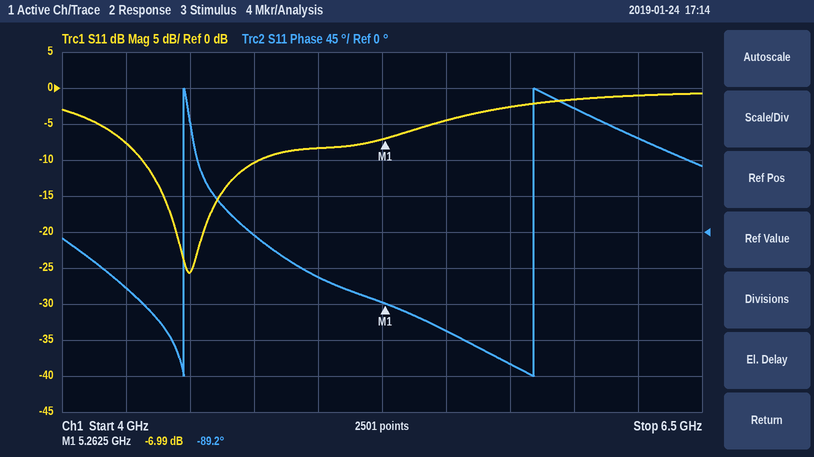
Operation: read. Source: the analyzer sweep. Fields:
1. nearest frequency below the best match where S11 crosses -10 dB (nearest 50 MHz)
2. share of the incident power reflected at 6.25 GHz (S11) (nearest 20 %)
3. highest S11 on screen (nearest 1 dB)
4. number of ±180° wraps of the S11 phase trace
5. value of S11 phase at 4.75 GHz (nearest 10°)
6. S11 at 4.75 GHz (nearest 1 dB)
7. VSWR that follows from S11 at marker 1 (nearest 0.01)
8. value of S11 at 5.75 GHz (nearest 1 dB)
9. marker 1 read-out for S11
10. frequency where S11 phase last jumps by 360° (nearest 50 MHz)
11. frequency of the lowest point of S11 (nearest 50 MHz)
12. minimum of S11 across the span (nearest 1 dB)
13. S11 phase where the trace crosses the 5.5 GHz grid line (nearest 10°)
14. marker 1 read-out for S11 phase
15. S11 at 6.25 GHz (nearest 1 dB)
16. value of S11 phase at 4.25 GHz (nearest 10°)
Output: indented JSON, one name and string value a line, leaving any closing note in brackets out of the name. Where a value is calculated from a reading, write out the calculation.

{
  "nearest frequency below the best match where S11 crosses -10 dB": "4.30 GHz",
  "share of the incident power reflected at 6.25 GHz (S11)": "10^(-1/10) ≈ 79.4 %, so 80 % to the nearest 20 %",
  "highest S11 on screen": "-1 dB",
  "number of ±180° wraps of the S11 phase trace": "2",
  "value of S11 phase at 4.75 GHz": "0°",
  "S11 at 4.75 GHz": "-10 dB",
  "VSWR that follows from S11 at marker 1": "(1 + 0.4472)/(1 − 0.4472) ≈ 2.62",
  "value of S11 at 5.75 GHz": "-3 dB",
  "marker 1 read-out for S11": "-6.99 dB",
  "frequency where S11 phase last jumps by 360°": "5.85 GHz",
  "frequency of the lowest point of S11": "4.50 GHz",
  "minimum of S11 across the span": "-26 dB",
  "S11 phase where the trace crosses the 5.5 GHz grid line": "-120°",
  "marker 1 read-out for S11 phase": "-89.2°",
  "S11 at 6.25 GHz": "-1 dB",
  "value of S11 phase at 4.25 GHz": "-70°"
}
